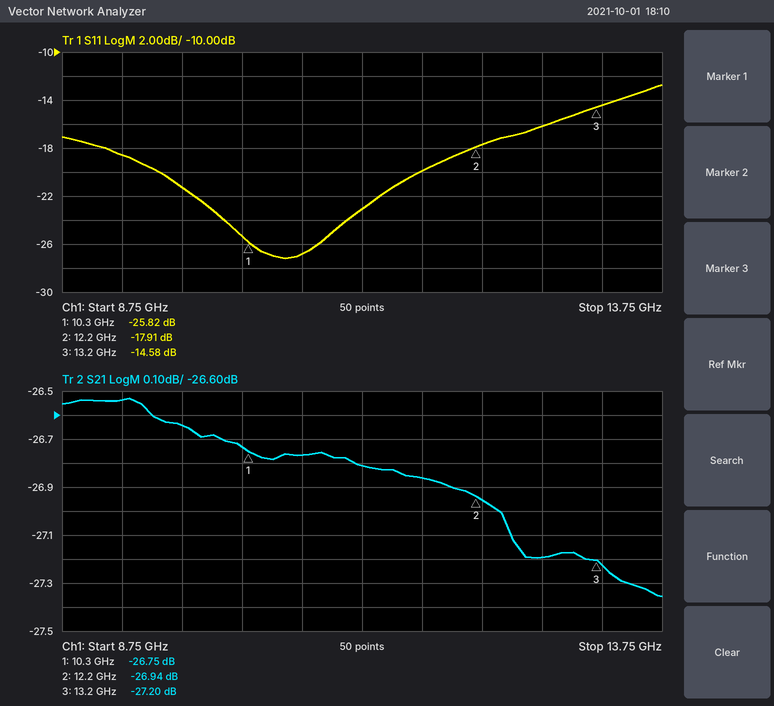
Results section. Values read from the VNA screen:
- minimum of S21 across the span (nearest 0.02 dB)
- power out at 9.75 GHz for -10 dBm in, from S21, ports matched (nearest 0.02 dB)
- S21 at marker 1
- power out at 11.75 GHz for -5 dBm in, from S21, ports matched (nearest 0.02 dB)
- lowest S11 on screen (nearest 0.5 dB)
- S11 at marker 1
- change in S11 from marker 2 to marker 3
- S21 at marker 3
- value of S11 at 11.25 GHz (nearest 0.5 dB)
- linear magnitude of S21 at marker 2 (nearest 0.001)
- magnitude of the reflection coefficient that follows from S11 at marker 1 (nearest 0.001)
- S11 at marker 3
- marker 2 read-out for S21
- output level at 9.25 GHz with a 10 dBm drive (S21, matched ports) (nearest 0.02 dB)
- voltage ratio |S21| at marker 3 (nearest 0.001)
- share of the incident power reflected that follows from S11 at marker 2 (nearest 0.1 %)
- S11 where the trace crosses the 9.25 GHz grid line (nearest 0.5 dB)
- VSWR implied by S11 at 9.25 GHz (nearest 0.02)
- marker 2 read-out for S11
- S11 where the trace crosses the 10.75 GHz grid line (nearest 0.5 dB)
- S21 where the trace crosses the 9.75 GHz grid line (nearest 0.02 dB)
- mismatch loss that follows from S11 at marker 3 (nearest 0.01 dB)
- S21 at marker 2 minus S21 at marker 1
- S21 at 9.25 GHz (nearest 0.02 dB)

-27.36 dB
-36.64 dBm
-26.75 dB
-31.86 dBm
-27.0 dB
-25.82 dB
3.33 dB
-27.20 dB
-23.0 dB
0.045
0.051
-14.58 dB
-26.94 dB
-16.54 dBm
0.044
1.6 %
-18.5 dB
1.26
-17.91 dB
-27.0 dB
-26.64 dB
0.15 dB
-0.19 dB
-26.54 dB
